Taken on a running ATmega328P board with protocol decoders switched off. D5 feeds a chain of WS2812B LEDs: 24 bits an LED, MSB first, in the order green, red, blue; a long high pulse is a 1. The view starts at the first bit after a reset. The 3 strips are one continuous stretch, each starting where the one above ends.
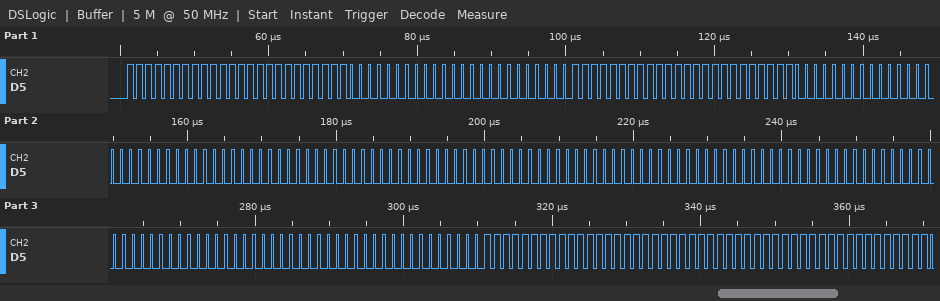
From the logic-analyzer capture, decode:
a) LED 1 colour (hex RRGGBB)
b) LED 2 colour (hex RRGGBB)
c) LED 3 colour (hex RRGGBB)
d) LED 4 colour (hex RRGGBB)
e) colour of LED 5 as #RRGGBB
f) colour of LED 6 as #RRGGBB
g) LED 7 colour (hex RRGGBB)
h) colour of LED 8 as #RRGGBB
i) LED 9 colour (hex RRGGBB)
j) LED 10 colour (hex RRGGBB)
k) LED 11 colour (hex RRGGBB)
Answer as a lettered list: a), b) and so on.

a) #FFFFFF
b) #000000
c) #FFFFFF
d) #000000
e) #000000
f) #000000
g) #000000
h) #000000
i) #000000
j) #FFFFFF
k) #FFFFFF
